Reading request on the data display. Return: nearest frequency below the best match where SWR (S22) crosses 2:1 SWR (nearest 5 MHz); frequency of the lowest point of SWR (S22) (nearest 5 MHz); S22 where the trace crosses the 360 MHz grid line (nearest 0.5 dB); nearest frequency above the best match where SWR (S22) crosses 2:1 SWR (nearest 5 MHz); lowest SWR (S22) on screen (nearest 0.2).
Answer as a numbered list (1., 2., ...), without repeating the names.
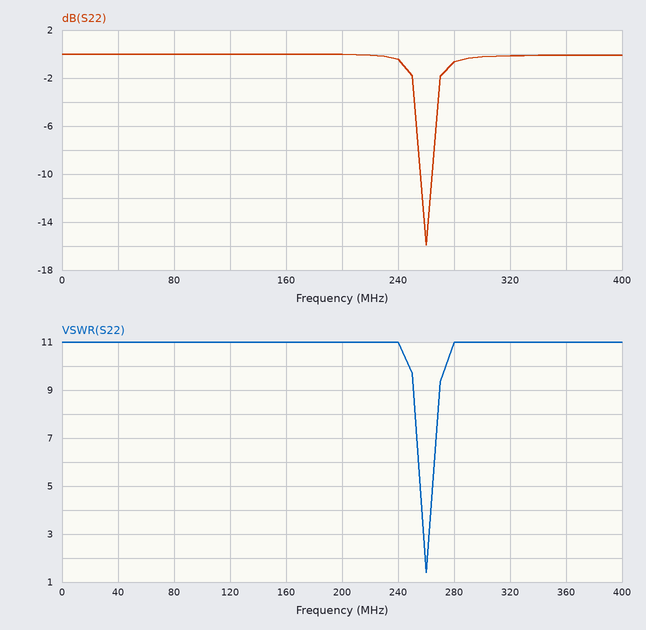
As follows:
1. 260 MHz
2. 260 MHz
3. 0.0 dB
4. 260 MHz
5. 1.4
